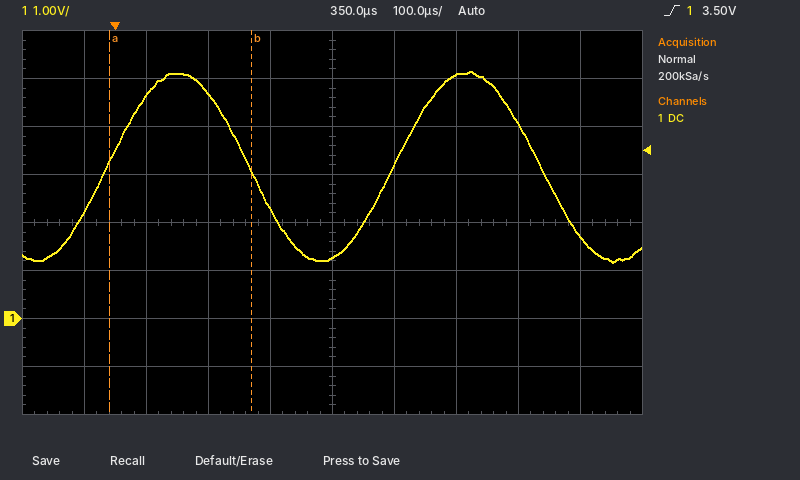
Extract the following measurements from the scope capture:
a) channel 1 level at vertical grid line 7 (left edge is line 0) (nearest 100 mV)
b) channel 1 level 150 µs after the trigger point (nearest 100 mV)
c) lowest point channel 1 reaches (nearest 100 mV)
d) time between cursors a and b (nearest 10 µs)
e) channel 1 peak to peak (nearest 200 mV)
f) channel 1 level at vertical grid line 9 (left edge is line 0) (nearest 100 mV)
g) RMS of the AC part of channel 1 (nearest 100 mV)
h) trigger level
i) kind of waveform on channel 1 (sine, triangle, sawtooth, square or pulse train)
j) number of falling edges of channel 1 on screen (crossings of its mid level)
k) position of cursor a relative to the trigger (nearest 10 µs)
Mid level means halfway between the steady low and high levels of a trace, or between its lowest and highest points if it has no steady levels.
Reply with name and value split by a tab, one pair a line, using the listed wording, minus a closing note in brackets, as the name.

channel 1 level at vertical grid line 7 (left edge is line 0)	5.1 V
channel 1 level 150 µs after the trigger point	4.7 V
lowest point channel 1 reaches	1.2 V
time between cursors a and b	230 µs
channel 1 peak to peak	4.0 V
channel 1 level at vertical grid line 9 (left edge is line 0)	1.7 V
RMS of the AC part of channel 1	1.4 V
trigger level	3.50 V
kind of waveform on channel 1	sine
number of falling edges of channel 1 on screen	2
position of cursor a relative to the trigger	-10 µs
